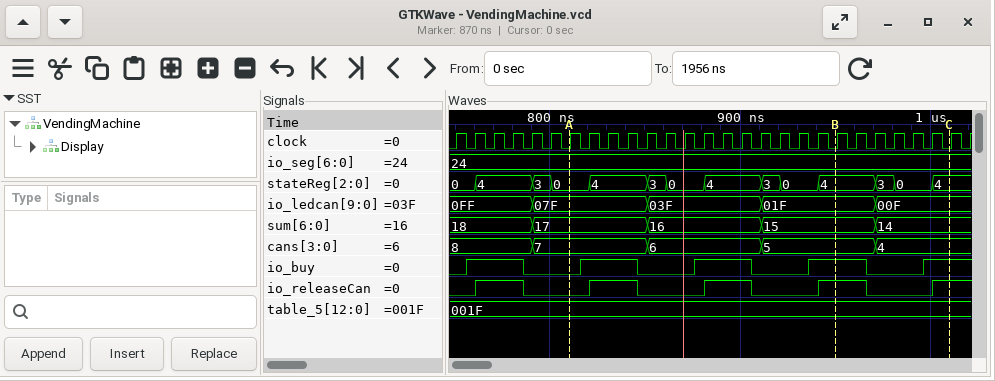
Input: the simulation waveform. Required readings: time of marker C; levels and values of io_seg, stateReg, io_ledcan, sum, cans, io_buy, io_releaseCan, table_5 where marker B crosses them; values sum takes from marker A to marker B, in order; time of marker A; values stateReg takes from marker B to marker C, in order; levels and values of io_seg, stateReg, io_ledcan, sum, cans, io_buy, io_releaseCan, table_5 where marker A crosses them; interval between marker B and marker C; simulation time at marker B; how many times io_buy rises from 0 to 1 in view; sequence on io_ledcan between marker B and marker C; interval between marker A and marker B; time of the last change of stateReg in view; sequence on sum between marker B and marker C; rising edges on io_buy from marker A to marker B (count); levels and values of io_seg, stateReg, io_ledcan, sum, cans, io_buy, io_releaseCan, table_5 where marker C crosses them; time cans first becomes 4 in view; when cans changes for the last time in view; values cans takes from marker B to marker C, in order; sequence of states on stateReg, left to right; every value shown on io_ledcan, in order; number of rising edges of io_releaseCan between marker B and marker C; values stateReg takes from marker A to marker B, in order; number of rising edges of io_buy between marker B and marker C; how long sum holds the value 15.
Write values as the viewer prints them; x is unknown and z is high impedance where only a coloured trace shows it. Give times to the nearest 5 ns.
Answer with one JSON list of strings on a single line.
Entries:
["1010 ns", "io_seg=24, stateReg=4, io_ledcan=01F, sum=15, cans=5, io_buy=1, io_releaseCan=1, table_5=001F", "17, 16, 15", "810 ns", "4, 3, 0, 4", "io_seg=24, stateReg=0, io_ledcan=07F, sum=17, cans=7, io_buy=0, io_releaseCan=0, table_5=001F", "60 ns", "950 ns", "5", "01F, 00F", "140 ns", "1000 ns", "15, 14", "3", "io_seg=24, stateReg=4, io_ledcan=00F, sum=14, cans=4, io_buy=1, io_releaseCan=1, table_5=001F", "970 ns", "970 ns", "5, 4", "0, 4, 3, 0, 4, 3, 0, 4, 3, 0, 4, 3, 0, 4", "0FF, 07F, 03F, 01F, 00F", "1", "0, 4, 3, 0, 4, 3, 0, 4", "1", "60 ns"]
